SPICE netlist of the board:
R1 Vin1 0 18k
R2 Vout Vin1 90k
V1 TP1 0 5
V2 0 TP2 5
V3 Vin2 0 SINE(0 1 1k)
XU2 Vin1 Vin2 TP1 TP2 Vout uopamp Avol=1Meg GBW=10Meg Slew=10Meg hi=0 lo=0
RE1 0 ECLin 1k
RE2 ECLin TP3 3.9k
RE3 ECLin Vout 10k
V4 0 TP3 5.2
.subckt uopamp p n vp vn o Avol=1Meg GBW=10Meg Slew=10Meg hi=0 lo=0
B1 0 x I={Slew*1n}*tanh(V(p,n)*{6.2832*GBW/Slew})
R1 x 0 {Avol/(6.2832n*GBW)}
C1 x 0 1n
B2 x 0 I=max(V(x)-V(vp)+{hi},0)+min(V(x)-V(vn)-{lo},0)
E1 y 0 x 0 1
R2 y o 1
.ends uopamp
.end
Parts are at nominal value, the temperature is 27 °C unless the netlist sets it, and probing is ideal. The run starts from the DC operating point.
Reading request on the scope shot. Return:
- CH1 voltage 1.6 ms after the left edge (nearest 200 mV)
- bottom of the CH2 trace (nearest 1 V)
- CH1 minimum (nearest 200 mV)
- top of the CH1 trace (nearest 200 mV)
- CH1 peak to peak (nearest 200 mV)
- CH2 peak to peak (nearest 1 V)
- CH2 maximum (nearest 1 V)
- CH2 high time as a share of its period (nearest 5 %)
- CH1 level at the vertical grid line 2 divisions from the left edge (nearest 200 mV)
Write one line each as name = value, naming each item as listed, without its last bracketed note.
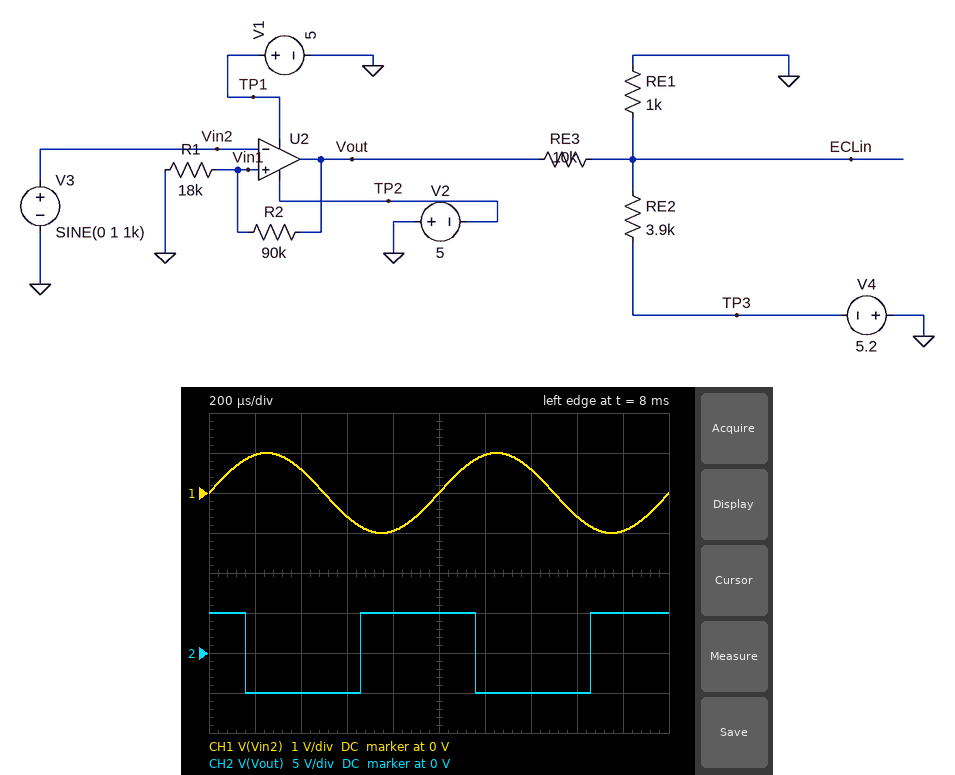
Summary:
CH1 voltage 1.6 ms after the left edge = -600 mV
bottom of the CH2 trace = -5 V
CH1 minimum = -1.0 V
top of the CH1 trace = 1.0 V
CH1 peak to peak = 2.0 V
CH2 peak to peak = 10 V
CH2 maximum = 5 V
CH2 high time as a share of its period = 50 %
CH1 level at the vertical grid line 2 divisions from the left edge = 600 mV
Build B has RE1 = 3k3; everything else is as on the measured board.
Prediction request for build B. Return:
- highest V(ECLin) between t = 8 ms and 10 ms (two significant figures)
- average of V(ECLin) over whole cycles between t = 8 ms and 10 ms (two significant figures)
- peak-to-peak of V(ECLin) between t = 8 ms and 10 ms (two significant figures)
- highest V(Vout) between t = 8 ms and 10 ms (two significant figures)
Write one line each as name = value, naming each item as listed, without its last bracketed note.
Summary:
highest V(ECLin) between t = 8 ms and 10 ms = -1.3 V
average of V(ECLin) over whole cycles between t = 8 ms and 10 ms = -2.0 V
peak-to-peak of V(ECLin) between t = 8 ms and 10 ms = 1.5 V
highest V(Vout) between t = 8 ms and 10 ms = 5.0 V
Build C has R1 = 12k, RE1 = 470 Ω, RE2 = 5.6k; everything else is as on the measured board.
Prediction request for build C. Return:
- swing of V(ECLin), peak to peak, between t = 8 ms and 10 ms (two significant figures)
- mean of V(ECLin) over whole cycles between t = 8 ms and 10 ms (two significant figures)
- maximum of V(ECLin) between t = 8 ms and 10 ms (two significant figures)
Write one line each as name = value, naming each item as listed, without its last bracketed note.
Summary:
swing of V(ECLin), peak to peak, between t = 8 ms and 10 ms = 420 mV
mean of V(ECLin) over whole cycles between t = 8 ms and 10 ms = -390 mV
maximum of V(ECLin) between t = 8 ms and 10 ms = -180 mV
